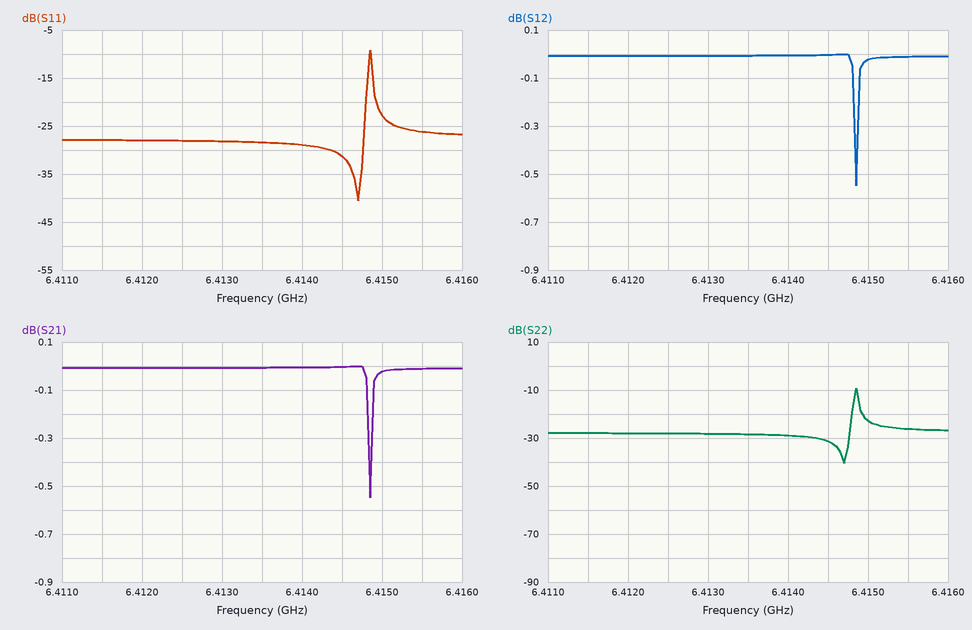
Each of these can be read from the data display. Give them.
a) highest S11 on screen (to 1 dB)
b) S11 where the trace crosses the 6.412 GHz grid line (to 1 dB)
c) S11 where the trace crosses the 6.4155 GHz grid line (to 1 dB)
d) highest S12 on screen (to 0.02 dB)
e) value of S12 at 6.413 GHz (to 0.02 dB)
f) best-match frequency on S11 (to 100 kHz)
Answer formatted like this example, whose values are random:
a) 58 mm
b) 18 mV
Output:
a) -9 dB
b) -28 dB
c) -26 dB
d) 0.00 dB
e) 0.00 dB
f) 6.4147 GHz
